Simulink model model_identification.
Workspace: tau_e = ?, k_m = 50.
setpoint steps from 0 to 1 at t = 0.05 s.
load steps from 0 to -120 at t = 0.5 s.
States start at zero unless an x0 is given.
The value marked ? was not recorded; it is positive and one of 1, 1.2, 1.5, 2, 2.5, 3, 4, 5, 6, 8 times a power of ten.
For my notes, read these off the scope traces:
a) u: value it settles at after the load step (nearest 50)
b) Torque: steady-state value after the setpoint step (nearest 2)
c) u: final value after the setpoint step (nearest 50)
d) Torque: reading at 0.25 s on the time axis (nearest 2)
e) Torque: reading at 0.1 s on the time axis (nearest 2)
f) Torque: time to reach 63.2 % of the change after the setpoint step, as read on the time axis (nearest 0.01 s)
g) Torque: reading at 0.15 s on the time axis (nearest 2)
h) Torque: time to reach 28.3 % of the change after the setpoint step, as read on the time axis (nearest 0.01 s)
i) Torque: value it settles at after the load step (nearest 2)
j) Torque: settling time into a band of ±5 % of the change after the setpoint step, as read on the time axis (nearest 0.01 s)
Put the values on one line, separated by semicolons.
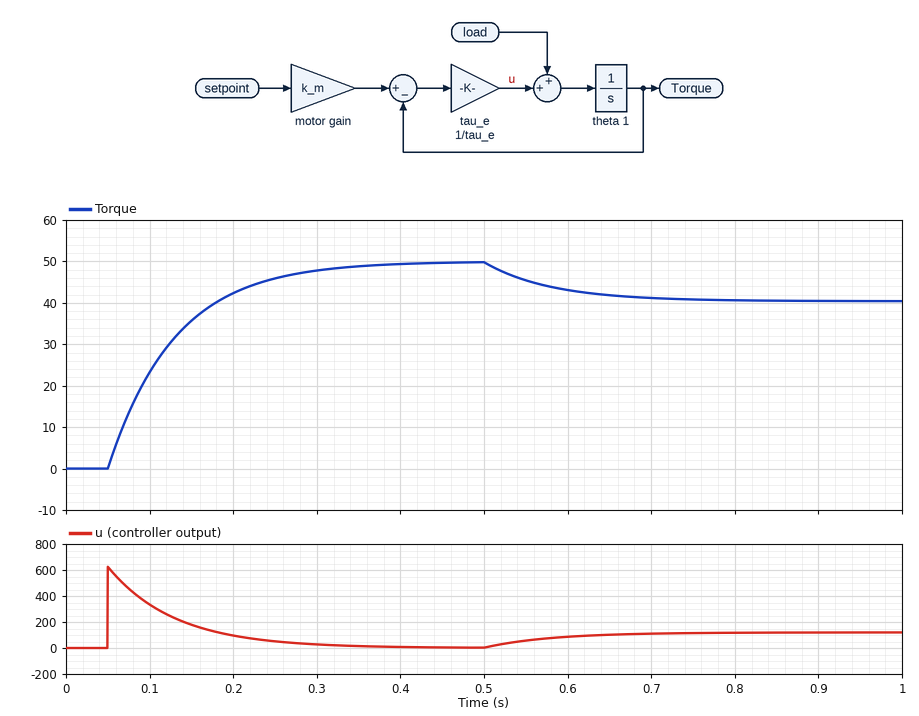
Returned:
100; 50; 0; 46; 24; 0.13 s; 36; 0.08 s; 40; 0.29 s
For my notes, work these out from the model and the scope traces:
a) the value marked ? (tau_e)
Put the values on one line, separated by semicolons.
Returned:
0.08
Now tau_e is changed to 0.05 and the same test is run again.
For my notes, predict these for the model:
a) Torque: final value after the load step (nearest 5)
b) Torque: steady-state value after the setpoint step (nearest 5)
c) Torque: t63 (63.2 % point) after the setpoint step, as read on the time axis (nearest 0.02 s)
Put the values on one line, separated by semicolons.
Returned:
45; 50; 0.10 s
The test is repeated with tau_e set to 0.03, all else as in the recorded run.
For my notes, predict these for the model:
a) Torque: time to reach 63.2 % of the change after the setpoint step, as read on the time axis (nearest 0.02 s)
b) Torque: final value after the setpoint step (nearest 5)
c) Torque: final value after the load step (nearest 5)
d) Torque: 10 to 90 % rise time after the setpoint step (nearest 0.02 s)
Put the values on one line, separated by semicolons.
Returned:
0.08 s; 50; 45; 0.06 s
